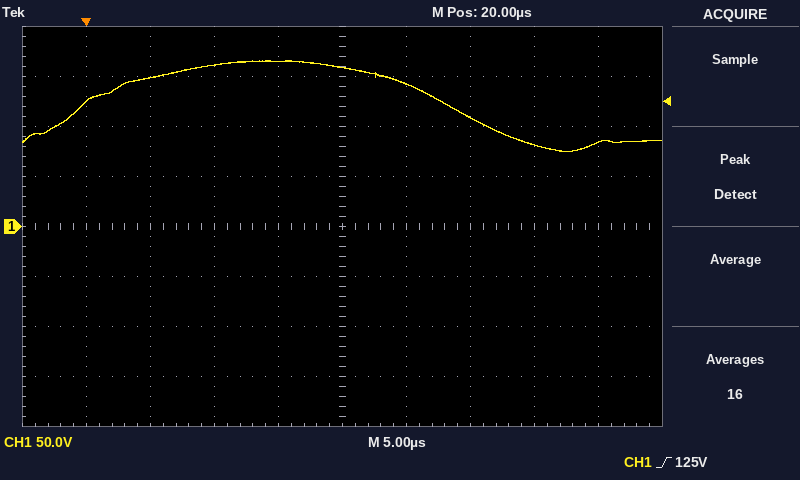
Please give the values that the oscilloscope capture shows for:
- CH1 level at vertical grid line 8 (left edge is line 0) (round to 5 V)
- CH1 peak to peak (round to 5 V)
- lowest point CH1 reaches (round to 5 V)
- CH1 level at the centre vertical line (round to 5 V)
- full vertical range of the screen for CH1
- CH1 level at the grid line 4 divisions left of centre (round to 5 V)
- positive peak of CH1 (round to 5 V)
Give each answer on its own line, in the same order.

80 V
90 V
75 V
160 V
400 V
125 V
165 V
